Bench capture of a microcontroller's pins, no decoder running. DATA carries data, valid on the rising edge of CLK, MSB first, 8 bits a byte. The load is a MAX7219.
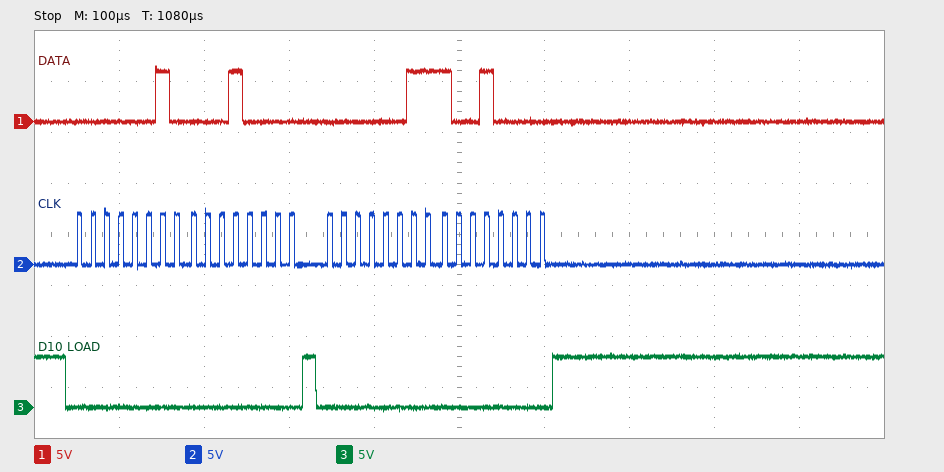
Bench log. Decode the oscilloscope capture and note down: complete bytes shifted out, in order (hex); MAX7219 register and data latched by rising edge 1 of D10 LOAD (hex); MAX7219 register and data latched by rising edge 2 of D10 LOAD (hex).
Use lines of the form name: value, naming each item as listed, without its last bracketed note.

complete bytes shifted out, in order: 02 10 03 90
MAX7219 register and data latched by rising edge 1 of D10 LOAD: register 0x2, data 0x10
MAX7219 register and data latched by rising edge 2 of D10 LOAD: register 0x3, data 0x90
